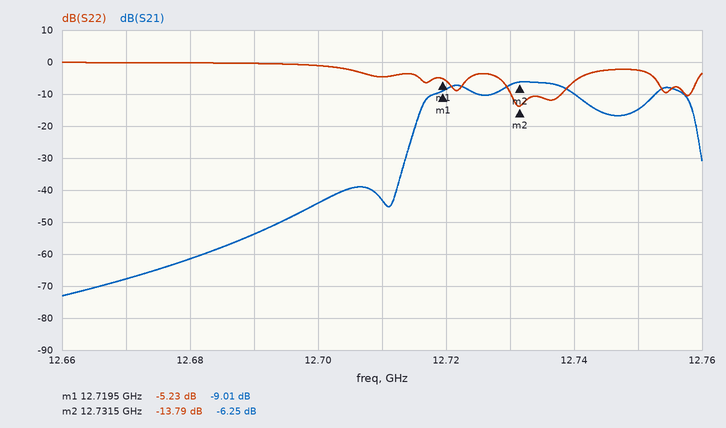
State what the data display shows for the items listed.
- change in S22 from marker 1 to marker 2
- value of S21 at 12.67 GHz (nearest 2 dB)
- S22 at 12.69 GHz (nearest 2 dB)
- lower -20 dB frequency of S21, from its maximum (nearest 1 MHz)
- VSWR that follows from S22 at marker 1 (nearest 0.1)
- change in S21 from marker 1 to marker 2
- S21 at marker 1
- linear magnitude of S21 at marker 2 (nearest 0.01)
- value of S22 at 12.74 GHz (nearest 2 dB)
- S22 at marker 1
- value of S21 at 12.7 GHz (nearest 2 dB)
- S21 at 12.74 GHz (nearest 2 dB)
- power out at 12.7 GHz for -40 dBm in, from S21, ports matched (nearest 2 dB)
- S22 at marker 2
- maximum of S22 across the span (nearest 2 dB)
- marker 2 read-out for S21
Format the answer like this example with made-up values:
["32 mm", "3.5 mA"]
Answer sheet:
["-8.56 dB", "-68 dB", "0 dB", "12.714 GHz", "3.4", "2.76 dB", "-9.01 dB", "0.49", "-6 dB", "-5.23 dB", "-44 dB", "-10 dB", "-84 dBm", "-13.79 dB", "0 dB", "-6.25 dB"]
